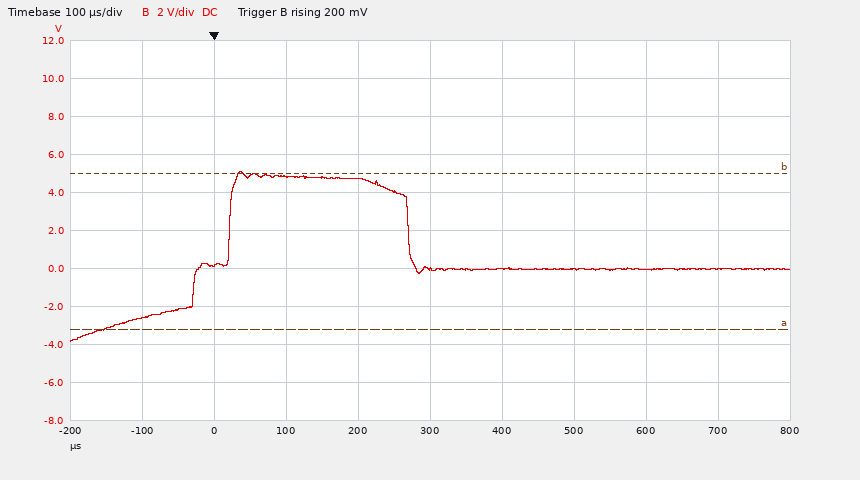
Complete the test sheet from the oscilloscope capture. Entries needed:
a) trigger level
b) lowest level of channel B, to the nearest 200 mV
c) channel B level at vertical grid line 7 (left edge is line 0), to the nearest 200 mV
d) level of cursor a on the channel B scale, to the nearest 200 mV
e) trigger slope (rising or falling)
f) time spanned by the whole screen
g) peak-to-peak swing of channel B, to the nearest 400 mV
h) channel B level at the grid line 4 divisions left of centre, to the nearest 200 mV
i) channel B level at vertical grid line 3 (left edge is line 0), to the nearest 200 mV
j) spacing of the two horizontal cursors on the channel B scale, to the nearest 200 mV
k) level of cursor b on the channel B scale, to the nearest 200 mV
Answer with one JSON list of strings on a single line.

["200 mV", "-3.8 V", "0.0 V", "-3.2 V", "rising", "1 ms", "8.8 V", "-2.6 V", "4.8 V", "8.2 V", "5.0 V"]
